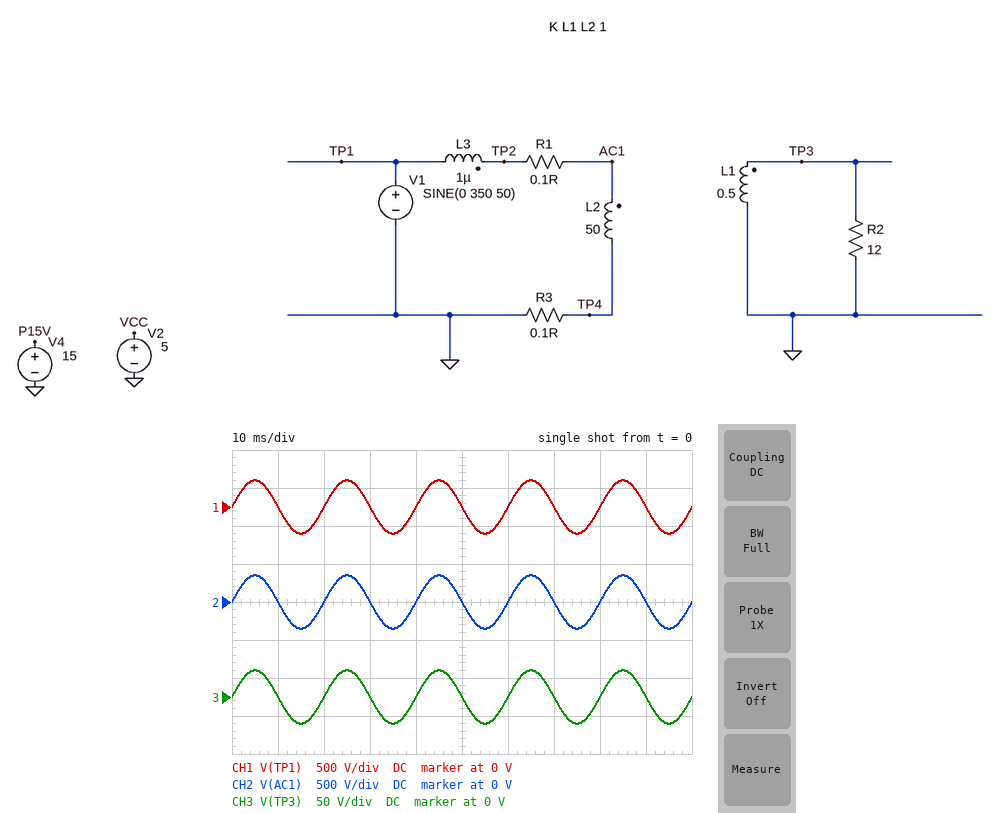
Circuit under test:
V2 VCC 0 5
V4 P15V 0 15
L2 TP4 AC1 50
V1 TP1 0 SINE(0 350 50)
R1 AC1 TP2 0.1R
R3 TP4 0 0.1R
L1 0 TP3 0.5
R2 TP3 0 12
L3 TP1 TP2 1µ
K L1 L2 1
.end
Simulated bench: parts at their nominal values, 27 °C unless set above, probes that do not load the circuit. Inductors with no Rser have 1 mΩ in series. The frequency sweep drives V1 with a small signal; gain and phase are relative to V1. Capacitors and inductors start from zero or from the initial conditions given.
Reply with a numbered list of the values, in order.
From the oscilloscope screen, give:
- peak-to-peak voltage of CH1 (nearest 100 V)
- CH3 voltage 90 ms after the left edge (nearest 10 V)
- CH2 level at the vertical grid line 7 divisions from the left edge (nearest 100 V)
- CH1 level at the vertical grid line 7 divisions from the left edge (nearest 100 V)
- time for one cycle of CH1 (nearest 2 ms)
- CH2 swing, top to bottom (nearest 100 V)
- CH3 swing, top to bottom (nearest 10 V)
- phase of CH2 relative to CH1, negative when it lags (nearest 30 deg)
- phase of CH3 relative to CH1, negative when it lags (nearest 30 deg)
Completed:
1. 700 V
2. 0 V
3. 0 V
4. 0 V
5. 20 ms
6. 700 V
7. 70 V
8. 0 deg
9. 0 deg
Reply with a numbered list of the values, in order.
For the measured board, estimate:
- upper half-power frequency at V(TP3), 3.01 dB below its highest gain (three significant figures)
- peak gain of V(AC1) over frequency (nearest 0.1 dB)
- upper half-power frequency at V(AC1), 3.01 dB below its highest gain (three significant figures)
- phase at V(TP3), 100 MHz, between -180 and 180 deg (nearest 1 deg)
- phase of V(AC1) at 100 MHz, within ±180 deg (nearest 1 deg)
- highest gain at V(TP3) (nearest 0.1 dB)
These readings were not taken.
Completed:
1. 191 MHz
2. 0 dB
3. 191 MHz
4. -28 deg
5. -28 deg
6. -20.0 dB
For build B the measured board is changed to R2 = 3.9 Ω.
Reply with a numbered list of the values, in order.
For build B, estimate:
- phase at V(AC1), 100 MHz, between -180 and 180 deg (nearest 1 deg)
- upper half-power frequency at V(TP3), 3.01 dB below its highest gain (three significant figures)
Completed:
1. -58 deg
2. 62.1 MHz
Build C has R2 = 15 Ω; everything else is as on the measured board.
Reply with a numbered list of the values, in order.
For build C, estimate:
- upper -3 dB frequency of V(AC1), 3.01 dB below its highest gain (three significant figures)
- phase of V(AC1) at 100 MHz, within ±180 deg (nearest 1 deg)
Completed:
1. 239 MHz
2. -23 deg
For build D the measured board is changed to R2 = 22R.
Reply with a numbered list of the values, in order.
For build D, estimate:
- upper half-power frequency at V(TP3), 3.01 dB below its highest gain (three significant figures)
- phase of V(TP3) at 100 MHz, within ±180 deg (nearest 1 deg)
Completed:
1. 350 MHz
2. -16 deg
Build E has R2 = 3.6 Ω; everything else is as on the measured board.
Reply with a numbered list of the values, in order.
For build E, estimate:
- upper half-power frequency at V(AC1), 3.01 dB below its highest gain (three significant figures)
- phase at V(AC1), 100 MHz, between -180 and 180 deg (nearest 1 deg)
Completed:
1. 57.3 MHz
2. -60 deg
